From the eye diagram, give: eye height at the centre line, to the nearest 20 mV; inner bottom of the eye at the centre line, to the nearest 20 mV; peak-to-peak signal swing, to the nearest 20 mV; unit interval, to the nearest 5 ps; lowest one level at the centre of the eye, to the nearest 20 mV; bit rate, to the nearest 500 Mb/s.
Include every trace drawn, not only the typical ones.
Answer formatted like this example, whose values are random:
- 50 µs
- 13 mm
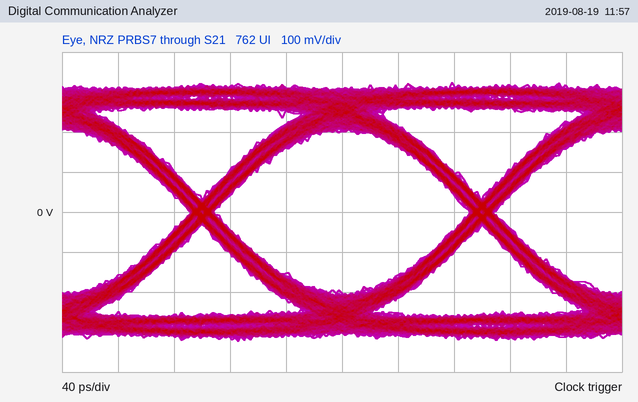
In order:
- 400 mV
- -200 mV
- 640 mV
- 200 ps
- 200 mV
- 5.0 Gb/s
